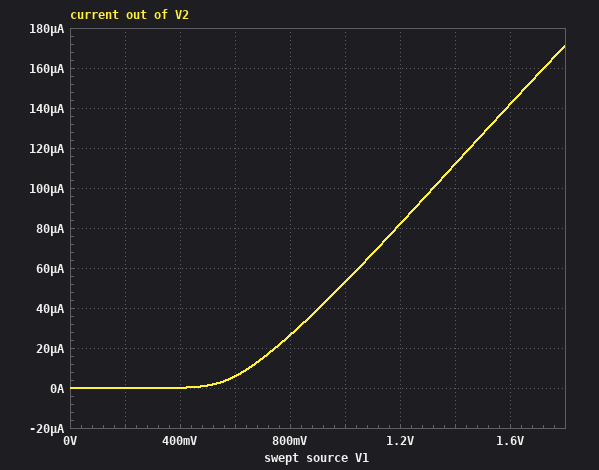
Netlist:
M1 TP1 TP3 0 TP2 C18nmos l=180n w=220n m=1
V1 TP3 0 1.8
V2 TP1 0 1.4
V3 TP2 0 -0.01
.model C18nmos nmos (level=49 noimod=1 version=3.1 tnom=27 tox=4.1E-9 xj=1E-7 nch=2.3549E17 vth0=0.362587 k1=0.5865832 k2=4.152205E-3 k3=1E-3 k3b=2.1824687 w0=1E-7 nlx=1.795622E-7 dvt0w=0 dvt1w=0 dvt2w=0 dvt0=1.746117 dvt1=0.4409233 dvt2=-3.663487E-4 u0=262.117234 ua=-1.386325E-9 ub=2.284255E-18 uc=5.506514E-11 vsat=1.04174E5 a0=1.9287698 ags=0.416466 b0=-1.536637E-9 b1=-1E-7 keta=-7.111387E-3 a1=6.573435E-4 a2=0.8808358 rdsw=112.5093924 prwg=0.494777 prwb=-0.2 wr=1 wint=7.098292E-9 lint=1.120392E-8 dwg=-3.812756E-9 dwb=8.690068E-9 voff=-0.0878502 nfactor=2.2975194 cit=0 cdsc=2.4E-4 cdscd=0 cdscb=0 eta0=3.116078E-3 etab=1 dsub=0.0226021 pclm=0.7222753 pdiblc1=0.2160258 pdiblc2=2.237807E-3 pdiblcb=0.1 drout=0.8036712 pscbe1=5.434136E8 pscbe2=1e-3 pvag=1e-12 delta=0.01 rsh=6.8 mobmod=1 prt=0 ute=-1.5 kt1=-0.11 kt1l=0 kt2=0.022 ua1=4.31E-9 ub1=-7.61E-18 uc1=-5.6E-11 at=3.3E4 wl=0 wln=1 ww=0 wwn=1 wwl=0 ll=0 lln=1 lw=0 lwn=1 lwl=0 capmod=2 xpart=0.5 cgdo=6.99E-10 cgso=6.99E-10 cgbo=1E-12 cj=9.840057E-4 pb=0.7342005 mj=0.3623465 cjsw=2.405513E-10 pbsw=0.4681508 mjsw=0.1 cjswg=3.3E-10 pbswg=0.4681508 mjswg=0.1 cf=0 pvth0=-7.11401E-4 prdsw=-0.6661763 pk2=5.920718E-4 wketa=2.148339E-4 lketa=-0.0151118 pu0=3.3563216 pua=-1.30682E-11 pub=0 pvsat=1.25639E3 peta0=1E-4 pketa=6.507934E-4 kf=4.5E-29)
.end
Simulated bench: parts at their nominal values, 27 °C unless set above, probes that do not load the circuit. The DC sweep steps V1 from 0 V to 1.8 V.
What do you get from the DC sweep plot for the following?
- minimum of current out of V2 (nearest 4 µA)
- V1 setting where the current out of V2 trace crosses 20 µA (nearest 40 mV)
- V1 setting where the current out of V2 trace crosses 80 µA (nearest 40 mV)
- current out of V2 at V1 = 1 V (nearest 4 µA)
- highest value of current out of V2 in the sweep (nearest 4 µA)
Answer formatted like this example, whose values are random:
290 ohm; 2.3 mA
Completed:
0 A; 760 mV; 1.20 V; 52 µA; 172 µA
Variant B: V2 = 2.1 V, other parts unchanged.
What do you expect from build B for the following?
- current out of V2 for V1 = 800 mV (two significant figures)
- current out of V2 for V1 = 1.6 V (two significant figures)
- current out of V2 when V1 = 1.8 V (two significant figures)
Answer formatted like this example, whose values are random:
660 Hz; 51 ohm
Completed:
42 µA; 160 µA; 180 µA
